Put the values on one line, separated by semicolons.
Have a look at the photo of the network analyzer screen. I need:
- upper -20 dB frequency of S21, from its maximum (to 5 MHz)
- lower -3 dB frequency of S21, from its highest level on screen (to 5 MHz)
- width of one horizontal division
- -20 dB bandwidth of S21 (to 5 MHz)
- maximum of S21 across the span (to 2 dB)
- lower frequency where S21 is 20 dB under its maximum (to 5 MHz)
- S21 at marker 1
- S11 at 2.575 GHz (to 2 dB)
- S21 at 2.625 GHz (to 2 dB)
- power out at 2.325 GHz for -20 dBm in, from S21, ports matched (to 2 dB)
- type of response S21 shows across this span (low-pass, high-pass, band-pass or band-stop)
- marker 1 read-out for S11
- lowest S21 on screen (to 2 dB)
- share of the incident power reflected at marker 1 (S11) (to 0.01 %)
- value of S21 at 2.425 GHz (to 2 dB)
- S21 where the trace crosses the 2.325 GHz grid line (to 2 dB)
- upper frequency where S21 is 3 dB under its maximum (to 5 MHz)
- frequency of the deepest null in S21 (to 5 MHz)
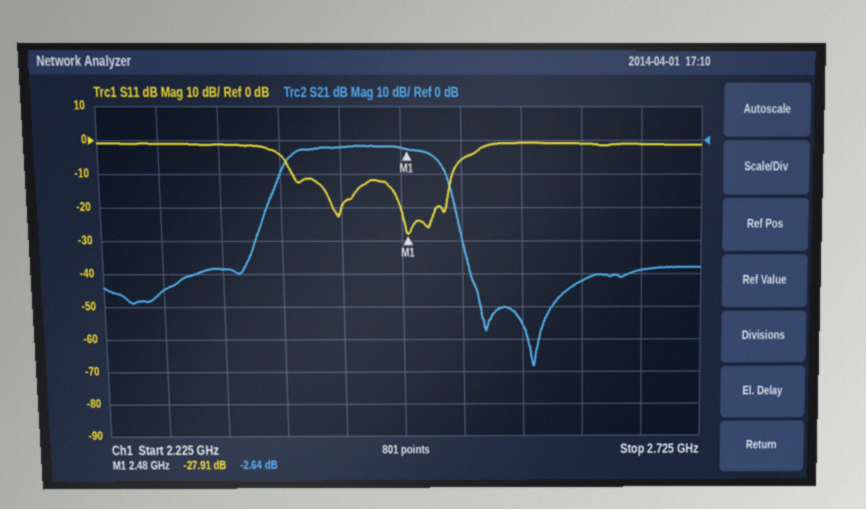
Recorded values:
2.520 GHz; 2.385 GHz; 50 MHz; 160 MHz; -2 dB; 2.360 GHz; -2.64 dB; 0 dB; -42 dB; -58 dBm; band-pass; -27.91 dB; -68 dB; 0.16 %; -2 dB; -38 dB; 2.500 GHz; 2.585 GHz
